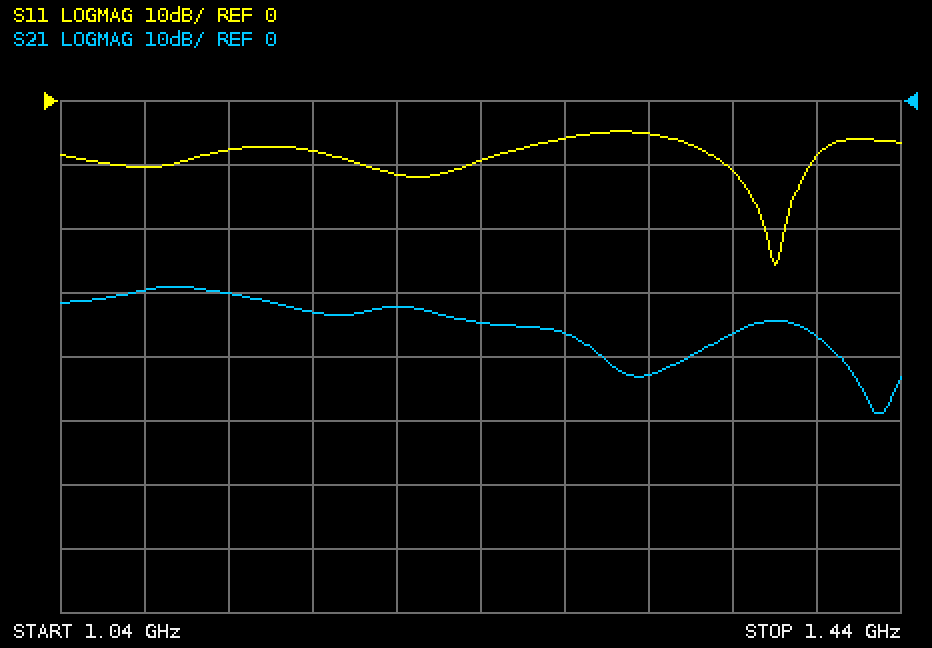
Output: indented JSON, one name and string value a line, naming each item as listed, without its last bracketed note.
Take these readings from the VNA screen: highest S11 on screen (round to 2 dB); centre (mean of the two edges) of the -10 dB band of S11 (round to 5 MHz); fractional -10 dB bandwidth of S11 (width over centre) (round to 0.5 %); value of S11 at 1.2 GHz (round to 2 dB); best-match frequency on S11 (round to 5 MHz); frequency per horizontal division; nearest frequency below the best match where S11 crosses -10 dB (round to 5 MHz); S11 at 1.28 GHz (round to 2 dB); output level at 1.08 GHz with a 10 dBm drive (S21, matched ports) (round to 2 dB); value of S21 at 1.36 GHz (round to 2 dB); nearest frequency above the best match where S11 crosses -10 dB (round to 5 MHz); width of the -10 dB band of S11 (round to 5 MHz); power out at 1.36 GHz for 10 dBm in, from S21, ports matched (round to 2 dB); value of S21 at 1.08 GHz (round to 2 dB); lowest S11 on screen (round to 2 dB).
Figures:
{
  "highest S11 on screen": "-4 dB",
  "centre (mean of the two edges) of the -10 dB band of S11": "1.375 GHz",
  "fractional -10 dB bandwidth of S11 (width over centre)": "3.0 %",
  "value of S11 at 1.2 GHz": "-12 dB",
  "best-match frequency on S11": "1.380 GHz",
  "frequency per horizontal division": "40 MHz",
  "nearest frequency below the best match where S11 crosses -10 dB": "1.355 GHz",
  "S11 at 1.28 GHz": "-6 dB",
  "output level at 1.08 GHz with a 10 dBm drive (S21, matched ports)": "-20 dBm",
  "value of S21 at 1.36 GHz": "-36 dB",
  "nearest frequency above the best match where S11 crosses -10 dB": "1.395 GHz",
  "width of the -10 dB band of S11": "40 MHz",
  "power out at 1.36 GHz for 10 dBm in, from S21, ports matched": "-26 dBm",
  "value of S21 at 1.08 GHz": "-30 dB",
  "lowest S11 on screen": "-26 dB"
}
